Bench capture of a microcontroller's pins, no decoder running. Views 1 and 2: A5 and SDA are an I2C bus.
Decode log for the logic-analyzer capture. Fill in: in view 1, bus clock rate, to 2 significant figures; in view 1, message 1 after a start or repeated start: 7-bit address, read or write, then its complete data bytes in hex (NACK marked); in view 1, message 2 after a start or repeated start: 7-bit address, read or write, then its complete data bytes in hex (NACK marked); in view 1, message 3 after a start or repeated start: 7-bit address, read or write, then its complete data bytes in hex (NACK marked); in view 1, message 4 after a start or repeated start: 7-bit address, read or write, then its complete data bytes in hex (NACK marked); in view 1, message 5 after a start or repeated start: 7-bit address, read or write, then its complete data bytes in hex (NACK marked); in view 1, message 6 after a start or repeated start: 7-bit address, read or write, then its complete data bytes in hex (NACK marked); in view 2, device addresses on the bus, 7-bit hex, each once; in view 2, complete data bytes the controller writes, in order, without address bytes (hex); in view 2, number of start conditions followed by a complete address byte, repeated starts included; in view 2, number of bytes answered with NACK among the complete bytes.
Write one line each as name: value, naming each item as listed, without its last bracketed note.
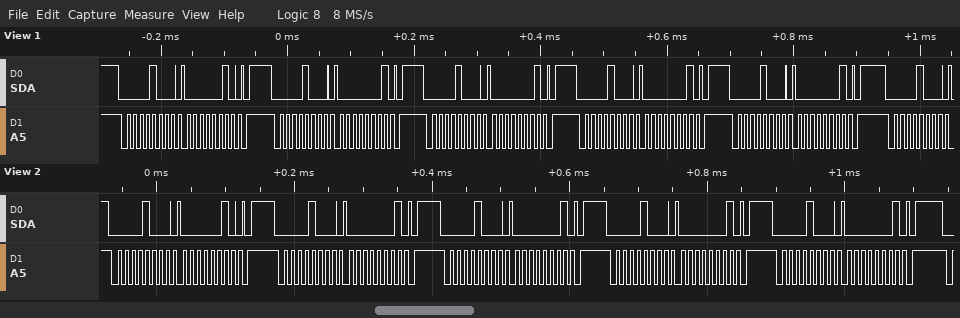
in view 1, bus clock rate, to 2 significant figures: 100 kHz
in view 1, message 1 after a start or repeated start: 7-bit address, read or write, then its complete data bytes in hex: 0x04 write: 02
in view 1, message 2 after a start or repeated start: 7-bit address, read or write, then its complete data bytes in hex: 0x04 write: 01
in view 1, message 3 after a start or repeated start: 7-bit address, read or write, then its complete data bytes in hex: 0x04 write: 01
in view 1, message 4 after a start or repeated start: 7-bit address, read or write, then its complete data bytes in hex: 0x04 write: 01
in view 1, message 5 after a start or repeated start: 7-bit address, read or write, then its complete data bytes in hex: 0x04 write: 01
in view 1, message 6 after a start or repeated start: 7-bit address, read or write, then its complete data bytes in hex: 0x04 write
in view 2, device addresses on the bus, 7-bit hex, each once: 0x04
in view 2, complete data bytes the controller writes, in order, without address bytes: 02 01 01 01 01
in view 2, number of start conditions followed by a complete address byte, repeated starts included: 5
in view 2, number of bytes answered with NACK among the complete bytes: 0
